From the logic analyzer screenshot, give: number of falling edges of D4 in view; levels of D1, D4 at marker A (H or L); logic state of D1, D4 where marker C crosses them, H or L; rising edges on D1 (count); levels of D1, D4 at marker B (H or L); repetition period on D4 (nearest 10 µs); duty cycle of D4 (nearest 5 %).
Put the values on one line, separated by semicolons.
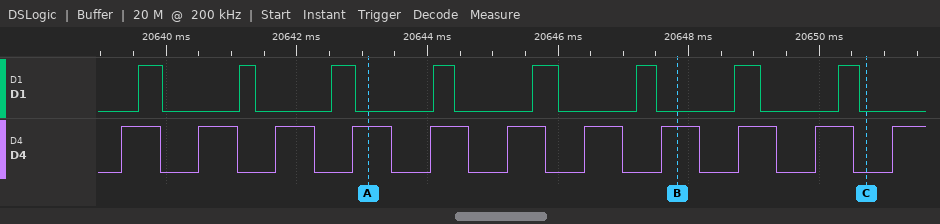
10; D1=L, D4=H; D1=L, D4=L; 8; D1=L, D4=H; 1180 µs; 50 %
